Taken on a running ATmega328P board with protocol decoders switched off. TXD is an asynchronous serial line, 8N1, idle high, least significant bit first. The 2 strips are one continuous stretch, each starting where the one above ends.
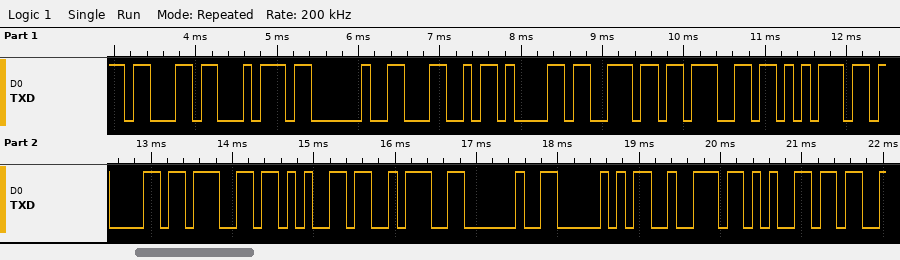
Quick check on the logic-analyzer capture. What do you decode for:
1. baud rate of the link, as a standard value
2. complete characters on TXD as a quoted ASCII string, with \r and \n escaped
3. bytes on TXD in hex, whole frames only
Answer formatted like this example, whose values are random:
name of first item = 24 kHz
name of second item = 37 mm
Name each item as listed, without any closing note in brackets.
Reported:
baud rate of the link, as a standard value = 9600 baud
complete characters on TXD as a quoted ASCII string, with \r and \n escaped = "ct Language: Pre"
bytes on TXD in hex, whole frames only = 63 74 20 4C 61 6E 67 75 61 67 65 3A 20 50 72 65
